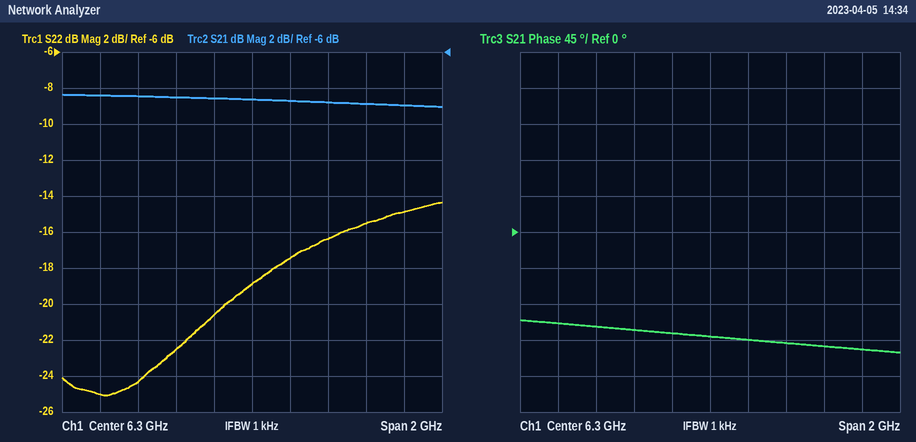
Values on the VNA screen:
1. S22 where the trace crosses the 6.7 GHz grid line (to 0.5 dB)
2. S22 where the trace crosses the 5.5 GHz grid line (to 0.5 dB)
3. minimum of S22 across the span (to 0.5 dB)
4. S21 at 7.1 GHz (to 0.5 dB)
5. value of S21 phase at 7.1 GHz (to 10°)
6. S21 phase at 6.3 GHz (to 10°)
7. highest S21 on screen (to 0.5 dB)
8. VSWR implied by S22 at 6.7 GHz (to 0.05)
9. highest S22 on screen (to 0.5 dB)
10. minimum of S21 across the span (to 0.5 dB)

-16.5 dB
-25.0 dB
-25.0 dB
-9.0 dB
-150°
-130°
-8.5 dB
1.35
-14.5 dB
-9.0 dB
